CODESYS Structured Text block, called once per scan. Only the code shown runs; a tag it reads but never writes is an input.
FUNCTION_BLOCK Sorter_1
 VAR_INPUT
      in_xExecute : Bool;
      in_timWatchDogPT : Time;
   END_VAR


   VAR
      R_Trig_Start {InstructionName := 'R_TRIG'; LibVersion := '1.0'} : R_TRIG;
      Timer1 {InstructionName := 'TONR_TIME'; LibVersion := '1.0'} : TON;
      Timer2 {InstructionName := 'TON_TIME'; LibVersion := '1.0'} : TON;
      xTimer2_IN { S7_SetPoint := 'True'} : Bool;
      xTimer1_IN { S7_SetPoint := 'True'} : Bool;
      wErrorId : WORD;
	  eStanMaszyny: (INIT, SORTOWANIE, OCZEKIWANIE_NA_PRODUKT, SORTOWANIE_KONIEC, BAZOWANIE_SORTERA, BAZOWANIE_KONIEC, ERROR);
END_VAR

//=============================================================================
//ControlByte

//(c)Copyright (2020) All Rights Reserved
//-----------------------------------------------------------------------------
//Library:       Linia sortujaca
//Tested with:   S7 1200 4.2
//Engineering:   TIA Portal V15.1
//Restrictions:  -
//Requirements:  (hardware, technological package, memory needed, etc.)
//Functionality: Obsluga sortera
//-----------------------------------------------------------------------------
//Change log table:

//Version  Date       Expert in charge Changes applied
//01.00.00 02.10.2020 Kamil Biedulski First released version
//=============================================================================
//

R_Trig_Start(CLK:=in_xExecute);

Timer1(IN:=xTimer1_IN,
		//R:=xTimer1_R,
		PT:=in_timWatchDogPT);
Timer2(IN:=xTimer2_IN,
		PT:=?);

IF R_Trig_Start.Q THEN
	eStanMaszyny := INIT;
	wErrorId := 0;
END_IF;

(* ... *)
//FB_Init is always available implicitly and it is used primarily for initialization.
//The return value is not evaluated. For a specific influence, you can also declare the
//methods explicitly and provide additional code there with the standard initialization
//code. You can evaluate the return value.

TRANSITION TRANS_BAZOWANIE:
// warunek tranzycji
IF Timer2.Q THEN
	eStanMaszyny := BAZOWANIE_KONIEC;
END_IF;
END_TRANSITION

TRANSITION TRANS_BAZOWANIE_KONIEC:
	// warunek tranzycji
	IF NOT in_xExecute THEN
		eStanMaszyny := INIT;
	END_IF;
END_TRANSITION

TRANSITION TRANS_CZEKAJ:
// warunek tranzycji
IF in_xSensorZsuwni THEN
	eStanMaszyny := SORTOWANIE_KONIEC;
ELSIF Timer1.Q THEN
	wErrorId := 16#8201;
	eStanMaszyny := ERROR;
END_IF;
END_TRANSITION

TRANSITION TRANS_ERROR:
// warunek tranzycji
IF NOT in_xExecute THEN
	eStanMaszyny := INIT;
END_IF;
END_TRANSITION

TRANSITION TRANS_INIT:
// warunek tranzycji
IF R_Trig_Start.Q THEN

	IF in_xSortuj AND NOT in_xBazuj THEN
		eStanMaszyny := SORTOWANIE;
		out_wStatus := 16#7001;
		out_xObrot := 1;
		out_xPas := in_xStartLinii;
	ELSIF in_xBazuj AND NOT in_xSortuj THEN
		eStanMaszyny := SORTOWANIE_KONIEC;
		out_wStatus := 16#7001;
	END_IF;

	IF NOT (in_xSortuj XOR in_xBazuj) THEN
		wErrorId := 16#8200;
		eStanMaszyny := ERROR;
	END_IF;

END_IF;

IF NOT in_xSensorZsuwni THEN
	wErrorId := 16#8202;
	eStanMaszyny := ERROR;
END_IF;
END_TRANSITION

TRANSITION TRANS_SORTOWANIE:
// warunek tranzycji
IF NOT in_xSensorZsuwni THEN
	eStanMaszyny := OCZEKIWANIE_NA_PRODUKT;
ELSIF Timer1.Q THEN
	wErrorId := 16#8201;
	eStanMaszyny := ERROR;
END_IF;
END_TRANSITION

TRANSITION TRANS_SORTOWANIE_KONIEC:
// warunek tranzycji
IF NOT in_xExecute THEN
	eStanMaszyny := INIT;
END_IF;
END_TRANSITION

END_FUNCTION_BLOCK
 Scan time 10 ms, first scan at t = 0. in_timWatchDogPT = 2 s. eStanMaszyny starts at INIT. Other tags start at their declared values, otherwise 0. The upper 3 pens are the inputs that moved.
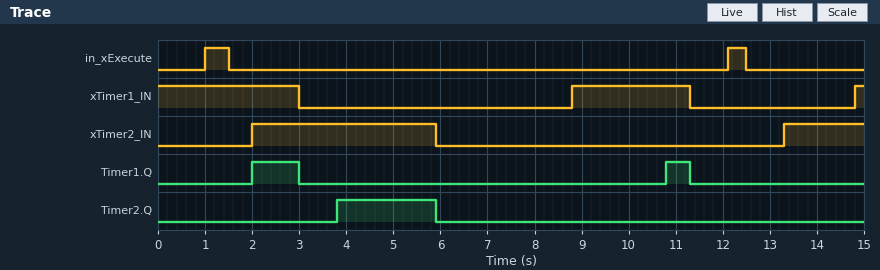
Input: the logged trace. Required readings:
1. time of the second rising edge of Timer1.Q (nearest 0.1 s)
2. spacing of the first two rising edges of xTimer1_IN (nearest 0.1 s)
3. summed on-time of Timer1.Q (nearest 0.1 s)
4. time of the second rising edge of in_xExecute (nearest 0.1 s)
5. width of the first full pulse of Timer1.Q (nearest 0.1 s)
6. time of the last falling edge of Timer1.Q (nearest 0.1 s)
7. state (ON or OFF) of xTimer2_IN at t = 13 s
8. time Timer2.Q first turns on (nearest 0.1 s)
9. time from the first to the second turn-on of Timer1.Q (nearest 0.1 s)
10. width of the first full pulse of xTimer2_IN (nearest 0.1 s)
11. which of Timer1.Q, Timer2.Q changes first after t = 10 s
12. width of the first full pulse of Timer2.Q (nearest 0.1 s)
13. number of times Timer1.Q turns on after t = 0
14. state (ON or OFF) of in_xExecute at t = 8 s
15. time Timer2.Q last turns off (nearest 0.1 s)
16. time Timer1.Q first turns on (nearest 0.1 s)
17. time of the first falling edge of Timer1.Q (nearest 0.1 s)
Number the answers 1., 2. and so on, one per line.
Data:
1. 10.8 s
2. 6.0 s
3. 1.5 s
4. 12.1 s
5. 1.0 s
6. 11.3 s
7. OFF
8. 3.8 s
9. 8.8 s
10. 3.9 s
11. Timer1.Q
12. 2.1 s
13. 2
14. OFF
15. 5.9 s
16. 2.0 s
17. 3.0 s
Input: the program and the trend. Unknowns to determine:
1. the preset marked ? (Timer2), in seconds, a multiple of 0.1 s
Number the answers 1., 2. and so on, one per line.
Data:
1. 1.8 s
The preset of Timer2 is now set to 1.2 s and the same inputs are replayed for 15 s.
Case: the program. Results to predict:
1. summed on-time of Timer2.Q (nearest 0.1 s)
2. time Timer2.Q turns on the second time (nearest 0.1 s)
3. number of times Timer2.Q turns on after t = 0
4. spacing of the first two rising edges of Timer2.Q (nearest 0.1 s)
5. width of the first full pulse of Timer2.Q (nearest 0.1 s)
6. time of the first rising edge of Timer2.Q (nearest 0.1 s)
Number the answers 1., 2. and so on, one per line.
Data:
1. 3.2 s
2. 14.5 s
3. 2
4. 11.3 s
5. 2.7 s
6. 3.2 s
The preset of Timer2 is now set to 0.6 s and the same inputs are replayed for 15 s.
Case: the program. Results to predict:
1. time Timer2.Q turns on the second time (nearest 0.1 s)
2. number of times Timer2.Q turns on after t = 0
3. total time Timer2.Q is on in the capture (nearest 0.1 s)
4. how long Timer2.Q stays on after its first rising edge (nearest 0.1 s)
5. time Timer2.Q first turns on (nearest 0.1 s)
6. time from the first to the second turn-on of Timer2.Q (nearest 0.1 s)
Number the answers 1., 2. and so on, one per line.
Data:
1. 13.9 s
2. 2
3. 4.4 s
4. 3.3 s
5. 2.6 s
6. 11.3 s
